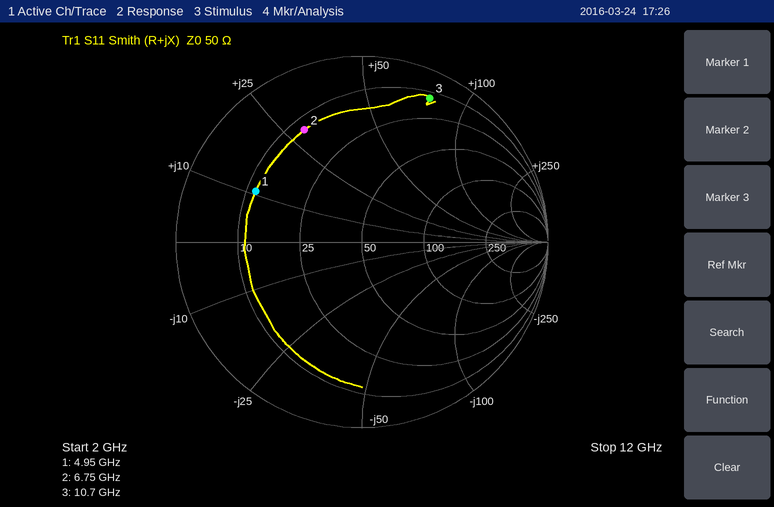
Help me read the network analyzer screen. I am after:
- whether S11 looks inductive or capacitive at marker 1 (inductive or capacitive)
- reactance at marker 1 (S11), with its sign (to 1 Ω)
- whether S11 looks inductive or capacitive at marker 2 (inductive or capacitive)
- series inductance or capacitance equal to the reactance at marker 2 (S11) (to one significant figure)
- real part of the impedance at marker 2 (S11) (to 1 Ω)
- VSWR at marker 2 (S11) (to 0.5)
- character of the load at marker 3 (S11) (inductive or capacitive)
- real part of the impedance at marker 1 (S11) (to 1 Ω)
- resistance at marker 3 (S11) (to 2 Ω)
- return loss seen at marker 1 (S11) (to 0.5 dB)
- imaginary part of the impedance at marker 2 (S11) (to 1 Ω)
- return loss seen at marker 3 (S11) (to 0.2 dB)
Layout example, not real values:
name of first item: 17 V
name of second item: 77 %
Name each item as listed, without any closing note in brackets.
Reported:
whether S11 looks inductive or capacitive at marker 1: inductive
reactance at marker 1 (S11), with its sign: +11 Ω
whether S11 looks inductive or capacitive at marker 2: inductive
series inductance or capacitance equal to the reactance at marker 2 (S11): 700 pH
real part of the impedance at marker 2 (S11): 13 Ω
VSWR at marker 2 (S11): 5.0
character of the load at marker 3 (S11): inductive
real part of the impedance at marker 1 (S11): 12 Ω
resistance at marker 3 (S11): 14 Ω
return loss seen at marker 1 (S11): 4.0 dB
imaginary part of the impedance at marker 2 (S11): +29 Ω
return loss seen at marker 3 (S11): 1.4 dB
